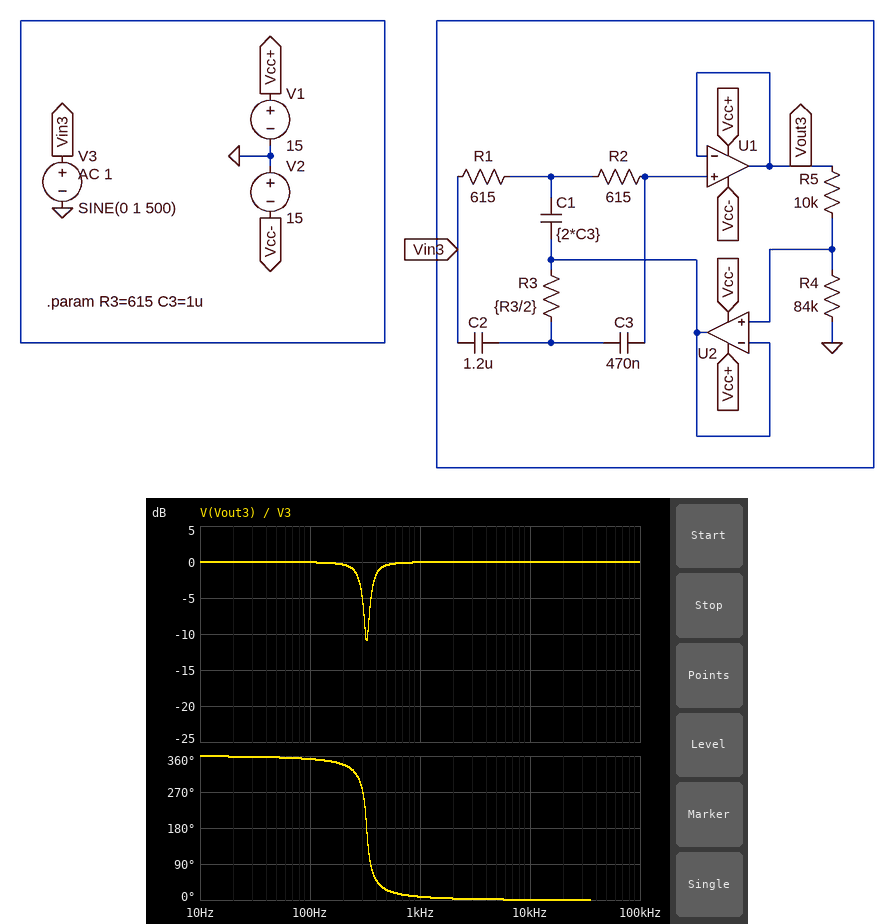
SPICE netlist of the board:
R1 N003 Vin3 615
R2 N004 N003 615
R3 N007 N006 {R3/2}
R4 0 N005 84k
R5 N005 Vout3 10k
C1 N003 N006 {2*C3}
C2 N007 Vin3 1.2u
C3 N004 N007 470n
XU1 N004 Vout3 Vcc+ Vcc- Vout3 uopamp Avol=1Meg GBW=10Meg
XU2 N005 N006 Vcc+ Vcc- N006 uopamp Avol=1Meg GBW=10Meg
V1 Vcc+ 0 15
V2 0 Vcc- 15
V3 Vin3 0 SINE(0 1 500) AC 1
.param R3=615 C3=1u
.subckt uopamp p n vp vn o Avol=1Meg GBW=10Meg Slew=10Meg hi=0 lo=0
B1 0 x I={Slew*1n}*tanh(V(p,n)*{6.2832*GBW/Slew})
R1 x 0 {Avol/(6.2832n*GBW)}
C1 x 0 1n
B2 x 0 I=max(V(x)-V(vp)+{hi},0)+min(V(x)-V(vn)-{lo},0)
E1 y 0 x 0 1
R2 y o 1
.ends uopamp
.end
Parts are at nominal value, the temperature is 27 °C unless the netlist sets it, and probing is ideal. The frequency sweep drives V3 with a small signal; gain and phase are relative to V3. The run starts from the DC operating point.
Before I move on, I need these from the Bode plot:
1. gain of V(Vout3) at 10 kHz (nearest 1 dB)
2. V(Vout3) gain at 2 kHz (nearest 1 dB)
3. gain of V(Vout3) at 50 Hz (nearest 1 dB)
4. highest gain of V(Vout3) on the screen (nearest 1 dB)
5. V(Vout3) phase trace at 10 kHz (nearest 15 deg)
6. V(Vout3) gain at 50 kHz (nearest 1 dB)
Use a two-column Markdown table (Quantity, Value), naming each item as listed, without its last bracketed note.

| Quantity | Value |
|---|---|
| gain of V(Vout3) at 10 kHz | 0 dB |
| V(Vout3) gain at 2 kHz | 0 dB |
| gain of V(Vout3) at 50 Hz | 0 dB |
| highest gain of V(Vout3) on the screen | 0 dB |
| V(Vout3) phase trace at 10 kHz | 0 deg |
| V(Vout3) gain at 50 kHz | 0 dB |
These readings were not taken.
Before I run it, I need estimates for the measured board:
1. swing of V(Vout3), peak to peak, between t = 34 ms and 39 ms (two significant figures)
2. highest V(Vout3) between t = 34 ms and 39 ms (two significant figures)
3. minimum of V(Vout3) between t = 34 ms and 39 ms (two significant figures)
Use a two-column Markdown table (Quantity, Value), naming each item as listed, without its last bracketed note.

| Quantity | Value |
|---|---|
| swing of V(Vout3), peak to peak, between t = 34 ms and 39 ms | 1.9 V |
| highest V(Vout3) between t = 34 ms and 39 ms | 950 mV |
| minimum of V(Vout3) between t = 34 ms and 39 ms | -950 mV |
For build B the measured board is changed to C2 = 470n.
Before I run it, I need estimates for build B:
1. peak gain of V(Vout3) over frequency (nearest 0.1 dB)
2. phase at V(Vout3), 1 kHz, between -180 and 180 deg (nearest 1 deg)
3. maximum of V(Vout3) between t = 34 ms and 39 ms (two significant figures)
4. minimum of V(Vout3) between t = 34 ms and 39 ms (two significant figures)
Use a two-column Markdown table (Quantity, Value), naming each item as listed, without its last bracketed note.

| Quantity | Value |
|---|---|
| peak gain of V(Vout3) over frequency | 3.0 dB |
| phase at V(Vout3), 1 kHz, between -180 and 180 deg | 17 deg |
| maximum of V(Vout3) between t = 34 ms and 39 ms | 1.2 V |
| minimum of V(Vout3) between t = 34 ms and 39 ms | -1.2 V |
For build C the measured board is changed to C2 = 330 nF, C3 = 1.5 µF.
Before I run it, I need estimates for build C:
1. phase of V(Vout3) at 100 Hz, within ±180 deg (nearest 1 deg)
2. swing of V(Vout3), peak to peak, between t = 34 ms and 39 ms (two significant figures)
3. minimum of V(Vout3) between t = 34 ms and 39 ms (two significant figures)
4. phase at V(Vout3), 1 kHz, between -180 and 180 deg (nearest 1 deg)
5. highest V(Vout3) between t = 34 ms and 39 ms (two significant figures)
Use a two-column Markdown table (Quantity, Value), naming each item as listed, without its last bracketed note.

| Quantity | Value |
|---|---|
| phase of V(Vout3) at 100 Hz, within ±180 deg | -13 deg |
| swing of V(Vout3), peak to peak, between t = 34 ms and 39 ms | 1.4 V |
| minimum of V(Vout3) between t = 34 ms and 39 ms | -690 mV |
| phase at V(Vout3), 1 kHz, between -180 and 180 deg | 17 deg |
| highest V(Vout3) between t = 34 ms and 39 ms | 690 mV |
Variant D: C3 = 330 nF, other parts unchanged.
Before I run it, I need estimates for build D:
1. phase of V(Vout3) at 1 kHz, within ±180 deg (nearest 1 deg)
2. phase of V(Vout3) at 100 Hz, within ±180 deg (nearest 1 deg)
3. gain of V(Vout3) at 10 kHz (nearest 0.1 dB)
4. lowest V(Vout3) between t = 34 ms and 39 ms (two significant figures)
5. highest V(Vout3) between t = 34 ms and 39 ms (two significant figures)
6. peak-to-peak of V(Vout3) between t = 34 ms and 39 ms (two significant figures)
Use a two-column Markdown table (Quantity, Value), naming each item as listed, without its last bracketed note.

| Quantity | Value |
|---|---|
| phase of V(Vout3) at 1 kHz, within ±180 deg | 10 deg |
| phase of V(Vout3) at 100 Hz, within ±180 deg | -7 deg |
| gain of V(Vout3) at 10 kHz | 0 dB |
| lowest V(Vout3) between t = 34 ms and 39 ms | -920 mV |
| highest V(Vout3) between t = 34 ms and 39 ms | 920 mV |
| peak-to-peak of V(Vout3) between t = 34 ms and 39 ms | 1.8 V |
